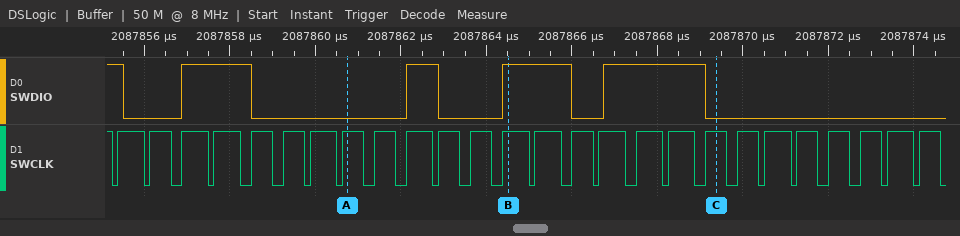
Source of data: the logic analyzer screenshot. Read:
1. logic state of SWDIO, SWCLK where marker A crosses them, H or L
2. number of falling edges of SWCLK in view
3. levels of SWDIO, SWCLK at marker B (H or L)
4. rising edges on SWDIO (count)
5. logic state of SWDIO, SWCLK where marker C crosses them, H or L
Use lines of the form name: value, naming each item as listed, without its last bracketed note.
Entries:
logic state of SWDIO, SWCLK where marker A crosses them, H or L: SWDIO=L, SWCLK=H
number of falling edges of SWCLK in view: 27
levels of SWDIO, SWCLK at marker B: SWDIO=H, SWCLK=H
rising edges on SWDIO: 4
logic state of SWDIO, SWCLK where marker C crosses them, H or L: SWDIO=L, SWCLK=H
